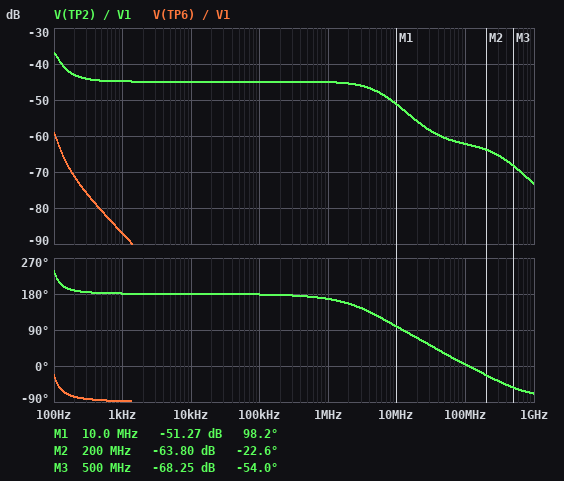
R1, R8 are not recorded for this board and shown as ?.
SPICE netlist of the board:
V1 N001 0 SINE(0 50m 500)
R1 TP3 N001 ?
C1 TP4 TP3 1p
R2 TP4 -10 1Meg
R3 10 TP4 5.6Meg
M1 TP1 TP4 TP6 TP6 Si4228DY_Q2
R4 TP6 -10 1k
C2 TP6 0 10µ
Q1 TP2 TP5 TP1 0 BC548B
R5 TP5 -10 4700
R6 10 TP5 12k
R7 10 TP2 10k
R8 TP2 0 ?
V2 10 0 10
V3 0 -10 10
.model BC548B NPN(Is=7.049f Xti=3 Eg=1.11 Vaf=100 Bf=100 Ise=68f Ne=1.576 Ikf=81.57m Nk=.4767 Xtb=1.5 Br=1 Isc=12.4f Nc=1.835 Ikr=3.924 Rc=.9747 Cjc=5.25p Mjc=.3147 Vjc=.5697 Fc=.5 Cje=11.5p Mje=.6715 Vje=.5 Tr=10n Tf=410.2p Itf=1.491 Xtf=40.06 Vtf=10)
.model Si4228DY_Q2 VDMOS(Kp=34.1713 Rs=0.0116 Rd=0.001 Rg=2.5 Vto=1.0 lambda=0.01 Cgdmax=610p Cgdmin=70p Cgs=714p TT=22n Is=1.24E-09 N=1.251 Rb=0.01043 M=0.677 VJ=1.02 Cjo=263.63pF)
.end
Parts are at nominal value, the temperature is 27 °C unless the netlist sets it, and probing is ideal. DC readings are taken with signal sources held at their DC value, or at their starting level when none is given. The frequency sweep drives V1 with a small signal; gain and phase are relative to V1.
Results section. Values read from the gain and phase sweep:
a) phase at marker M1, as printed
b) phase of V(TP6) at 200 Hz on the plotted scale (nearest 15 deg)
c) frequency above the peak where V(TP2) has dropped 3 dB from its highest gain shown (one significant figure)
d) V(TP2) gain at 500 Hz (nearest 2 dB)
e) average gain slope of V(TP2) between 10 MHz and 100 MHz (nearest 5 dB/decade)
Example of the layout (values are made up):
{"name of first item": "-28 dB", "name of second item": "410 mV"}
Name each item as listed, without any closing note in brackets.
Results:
{"phase at marker M1, as printed": "98.2 deg", "phase of V(TP6) at 200 Hz on the plotted scale": "-75 deg", "frequency above the peak where V(TP2) has dropped 3 dB from its highest gain shown": "100 Hz", "V(TP2) gain at 500 Hz": "-44 dB", "average gain slope of V(TP2) between 10 MHz and 100 MHz": "-10 dB/decade"}
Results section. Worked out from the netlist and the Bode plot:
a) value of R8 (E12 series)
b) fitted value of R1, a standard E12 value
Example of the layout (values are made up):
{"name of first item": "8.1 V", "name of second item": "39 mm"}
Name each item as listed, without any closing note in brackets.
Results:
{"value of R8": "8.2 kΩ", "fitted value of R1, a standard E12 value": "560 Ω"}
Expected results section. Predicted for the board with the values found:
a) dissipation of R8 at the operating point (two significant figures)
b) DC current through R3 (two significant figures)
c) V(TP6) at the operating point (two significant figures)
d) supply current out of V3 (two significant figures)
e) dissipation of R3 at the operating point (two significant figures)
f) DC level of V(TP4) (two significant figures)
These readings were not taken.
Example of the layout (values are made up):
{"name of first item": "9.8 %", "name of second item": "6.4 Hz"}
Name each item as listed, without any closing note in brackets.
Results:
{"dissipation of R8 at the operating point": "3.3 mW", "DC current through R3": "3.0 µA", "V(TP6) at the operating point": "-7.8 V", "supply current out of V3": "3.4 mA", "dissipation of R3 at the operating point": "51 µW", "DC level of V(TP4)": "-7.0 V"}
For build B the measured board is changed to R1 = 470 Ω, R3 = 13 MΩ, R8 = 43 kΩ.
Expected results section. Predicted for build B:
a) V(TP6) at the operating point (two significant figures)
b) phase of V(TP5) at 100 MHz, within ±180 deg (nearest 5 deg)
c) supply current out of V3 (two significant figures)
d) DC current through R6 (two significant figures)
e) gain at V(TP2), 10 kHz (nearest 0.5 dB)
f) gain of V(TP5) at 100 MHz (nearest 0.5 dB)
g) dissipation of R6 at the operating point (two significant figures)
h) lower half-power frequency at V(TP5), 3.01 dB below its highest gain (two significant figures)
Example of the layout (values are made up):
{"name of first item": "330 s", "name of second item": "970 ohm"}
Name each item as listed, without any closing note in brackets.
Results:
{"V(TP6) at the operating point": "-9.3 V", "phase of V(TP5) at 100 MHz, within ±180 deg": "-5 deg", "supply current out of V3": "1.9 mA", "DC current through R6": "1.2 mA", "gain at V(TP2), 10 kHz": "-19.0 dB", "gain of V(TP5) at 100 MHz": "-62.5 dB", "dissipation of R6 at the operating point": "17 mW", "lower half-power frequency at V(TP5), 3.01 dB below its highest gain": "720 kHz"}
